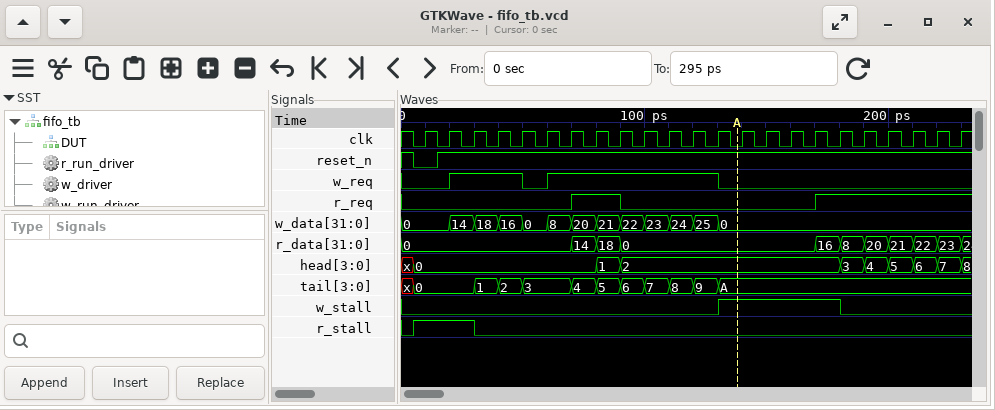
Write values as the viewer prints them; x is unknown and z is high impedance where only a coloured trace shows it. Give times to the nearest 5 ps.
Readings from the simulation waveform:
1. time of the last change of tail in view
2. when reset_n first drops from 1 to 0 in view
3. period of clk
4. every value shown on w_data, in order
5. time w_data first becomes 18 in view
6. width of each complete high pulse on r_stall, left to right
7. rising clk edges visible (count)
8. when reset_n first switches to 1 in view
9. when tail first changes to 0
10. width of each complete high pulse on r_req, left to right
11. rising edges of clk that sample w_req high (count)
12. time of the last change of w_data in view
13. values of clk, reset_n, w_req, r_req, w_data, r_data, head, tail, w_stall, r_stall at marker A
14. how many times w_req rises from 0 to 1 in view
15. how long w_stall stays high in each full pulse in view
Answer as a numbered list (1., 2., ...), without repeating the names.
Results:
1. 130 ps
2. 5 ps
3. 10 ps
4. 0, 14, 18, 16, 0, 8, 20, 21, 22, 23, 24, 25, 0
5. 30 ps
6. 25 ps
7. 23
8. 15 ps
9. 5 ps
10. 20 ps
11. 10
12. 130 ps
13. clk=0, reset_n=1, w_req=0, r_req=0, w_data=0, r_data=0, head=2, tail=A, w_stall=1, r_stall=0
14. 2
15. 50 ps
